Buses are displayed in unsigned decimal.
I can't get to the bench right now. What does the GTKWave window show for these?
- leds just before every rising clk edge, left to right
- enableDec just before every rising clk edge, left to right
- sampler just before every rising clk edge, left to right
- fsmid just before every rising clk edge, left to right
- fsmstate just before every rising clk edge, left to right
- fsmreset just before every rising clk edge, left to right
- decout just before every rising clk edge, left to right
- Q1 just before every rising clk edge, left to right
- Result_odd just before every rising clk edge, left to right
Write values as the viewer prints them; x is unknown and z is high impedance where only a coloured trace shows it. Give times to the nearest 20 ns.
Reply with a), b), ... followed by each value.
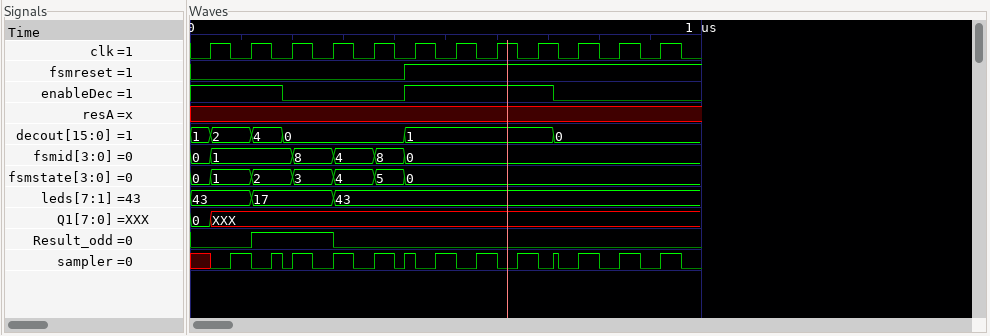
a) 43, 43, 17, 17, 43, 43, 43, 43, 43, 43, 43, 43
b) 1 1 0 0 0 1 1 1 1 0 0 0
c) x 1 0 0 0 1 1 1 1 0 0 0
d) 0, 1, 1, 8, 4, 0, 0, 0, 0, 0, 0, 0
e) 0, 1, 2, 3, 4, 0, 0, 0, 0, 0, 0, 0
f) 0 0 0 0 0 1 1 1 1 1 1 1
g) 1, 2, 0, 0, 0, 1, 1, 1, 1, 0, 0, 0
h) 0, XXX, XXX, XXX, XXX, XXX, XXX, XXX, XXX, XXX, XXX, XXX
i) 0 0 1 1 0 0 0 0 0 0 0 0
